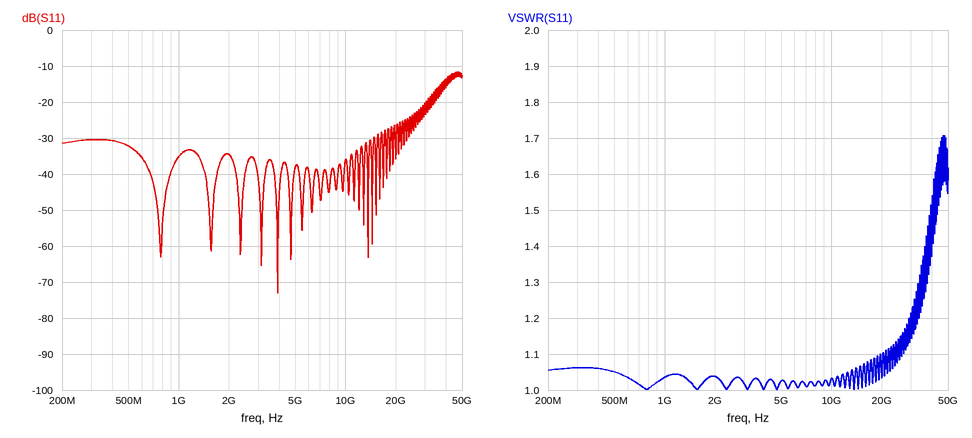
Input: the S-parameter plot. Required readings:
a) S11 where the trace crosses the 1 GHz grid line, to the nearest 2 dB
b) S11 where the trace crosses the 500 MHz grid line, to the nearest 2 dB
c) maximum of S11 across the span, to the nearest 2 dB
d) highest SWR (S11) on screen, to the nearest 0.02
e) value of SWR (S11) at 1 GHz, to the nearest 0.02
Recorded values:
-36 dB
-32 dB
-12 dB
1.70
1.04
